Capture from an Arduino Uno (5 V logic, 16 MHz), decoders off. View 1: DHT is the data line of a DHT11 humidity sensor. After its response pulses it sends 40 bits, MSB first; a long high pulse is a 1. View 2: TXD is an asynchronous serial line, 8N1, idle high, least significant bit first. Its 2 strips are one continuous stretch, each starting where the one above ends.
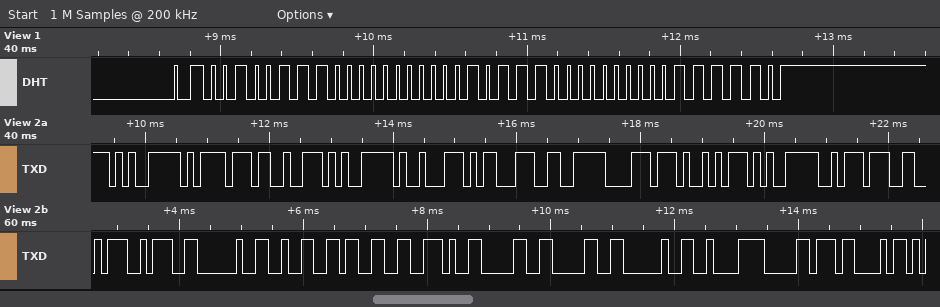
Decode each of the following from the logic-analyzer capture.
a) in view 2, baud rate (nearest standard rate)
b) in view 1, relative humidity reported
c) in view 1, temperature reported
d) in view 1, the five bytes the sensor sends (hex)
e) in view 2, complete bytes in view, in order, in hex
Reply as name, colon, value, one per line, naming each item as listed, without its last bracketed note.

in view 2, baud rate: 9600 baud
in view 1, relative humidity reported: 39 %
in view 1, temperature reported: 23.0 °C
in view 1, the five bytes the sensor sends: 27 00 17 00 3E
in view 2, complete bytes in view, in order, in hex: E5 BD 93 E5 89 8D E6 B8 A9 E5 BA A6 3A 20 32 33 2E 30 30 20 C2 B0 43
